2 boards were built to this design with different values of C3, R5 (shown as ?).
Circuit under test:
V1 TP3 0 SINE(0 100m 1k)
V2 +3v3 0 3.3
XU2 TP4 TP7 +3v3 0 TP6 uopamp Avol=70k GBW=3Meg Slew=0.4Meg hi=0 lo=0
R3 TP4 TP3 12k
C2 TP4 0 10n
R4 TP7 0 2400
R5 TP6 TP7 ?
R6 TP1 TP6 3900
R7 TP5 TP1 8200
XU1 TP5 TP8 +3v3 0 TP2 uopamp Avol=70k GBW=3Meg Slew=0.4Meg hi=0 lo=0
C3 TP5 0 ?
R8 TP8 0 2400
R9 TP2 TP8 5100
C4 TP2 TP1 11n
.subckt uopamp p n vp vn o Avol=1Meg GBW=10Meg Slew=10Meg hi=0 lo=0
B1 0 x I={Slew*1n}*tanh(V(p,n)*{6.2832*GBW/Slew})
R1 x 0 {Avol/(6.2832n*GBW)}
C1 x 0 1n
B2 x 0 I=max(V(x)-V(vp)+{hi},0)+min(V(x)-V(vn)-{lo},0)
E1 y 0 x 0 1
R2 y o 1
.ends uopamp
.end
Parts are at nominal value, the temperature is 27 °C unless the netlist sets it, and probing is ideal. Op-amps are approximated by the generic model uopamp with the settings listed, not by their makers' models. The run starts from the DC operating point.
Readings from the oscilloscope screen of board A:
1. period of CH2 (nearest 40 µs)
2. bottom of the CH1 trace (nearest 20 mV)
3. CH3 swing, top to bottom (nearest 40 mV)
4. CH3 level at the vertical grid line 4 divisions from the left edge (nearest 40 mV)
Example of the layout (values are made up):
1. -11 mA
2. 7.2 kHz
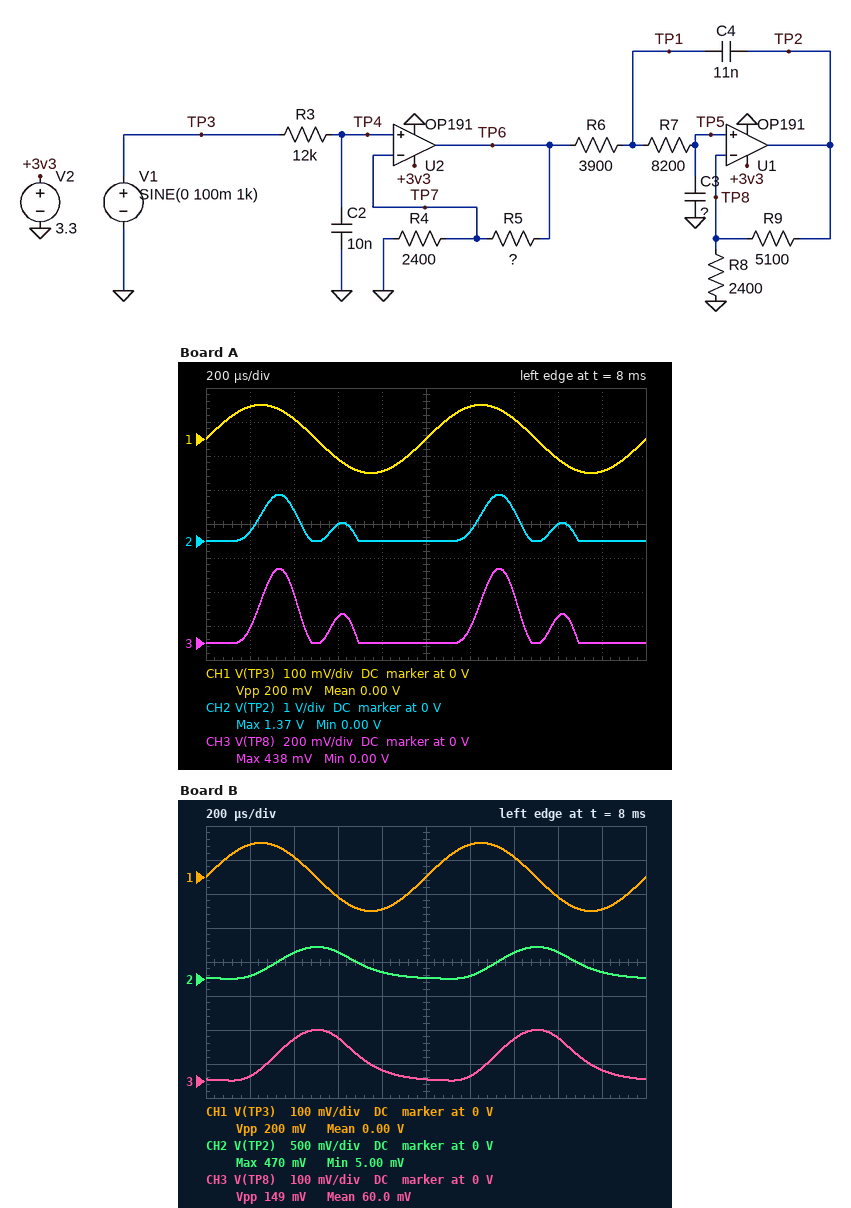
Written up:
1. 1.00 ms
2. -100 mV
3. 440 mV
4. 0 V
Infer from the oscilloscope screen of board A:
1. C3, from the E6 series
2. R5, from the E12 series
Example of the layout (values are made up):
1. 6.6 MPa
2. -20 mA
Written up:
1. 6.8 nF
2. 5.6 kΩ
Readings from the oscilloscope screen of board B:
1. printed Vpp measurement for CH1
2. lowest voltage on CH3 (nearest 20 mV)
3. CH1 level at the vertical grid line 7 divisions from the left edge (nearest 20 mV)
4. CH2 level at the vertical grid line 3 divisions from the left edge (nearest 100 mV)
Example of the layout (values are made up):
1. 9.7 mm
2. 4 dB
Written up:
1. 200 mV
2. 0 V
3. 60 mV
4. 400 mV
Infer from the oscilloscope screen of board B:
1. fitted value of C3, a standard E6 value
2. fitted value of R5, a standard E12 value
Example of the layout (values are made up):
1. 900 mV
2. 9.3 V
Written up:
1. 22 nF
2. 3.3 kΩ
